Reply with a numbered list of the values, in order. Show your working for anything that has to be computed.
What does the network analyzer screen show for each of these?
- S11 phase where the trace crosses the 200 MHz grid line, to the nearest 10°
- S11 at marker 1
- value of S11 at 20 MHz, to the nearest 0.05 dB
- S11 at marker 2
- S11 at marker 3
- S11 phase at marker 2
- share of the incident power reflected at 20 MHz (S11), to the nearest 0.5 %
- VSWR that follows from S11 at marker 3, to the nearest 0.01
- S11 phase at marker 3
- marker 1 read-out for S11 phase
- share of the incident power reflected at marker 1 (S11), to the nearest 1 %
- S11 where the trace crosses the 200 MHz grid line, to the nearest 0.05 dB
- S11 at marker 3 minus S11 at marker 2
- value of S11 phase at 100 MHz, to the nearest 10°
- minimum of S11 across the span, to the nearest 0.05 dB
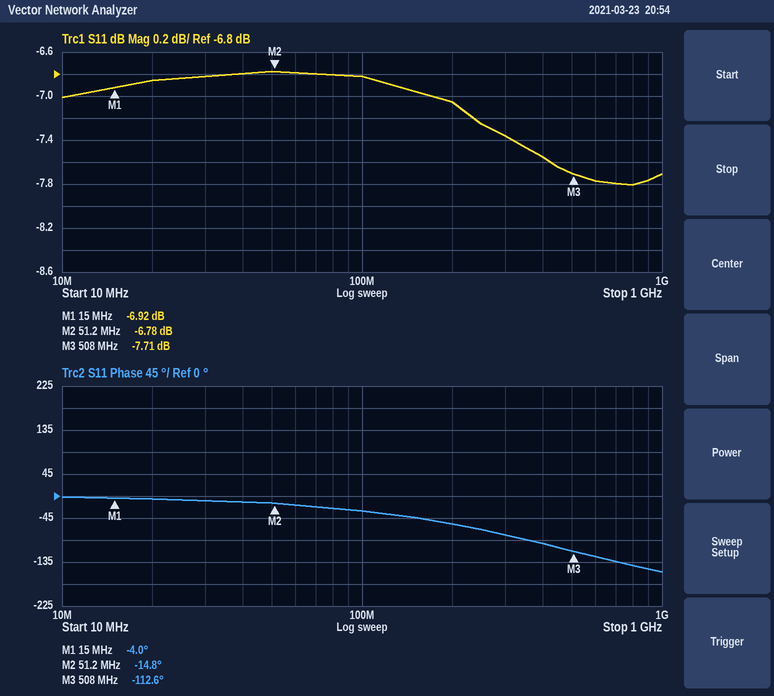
1. -60°
2. -6.92 dB
3. -6.85 dB
4. -6.78 dB
5. -7.71 dB
6. -14.8°
7. 10^(-6.85/10) ≈ 20.7 %, so 20.5 % to the nearest 0.5 %
8. (1 + 0.4116)/(1 − 0.4116) ≈ 2.40
9. -112.6°
10. -4.0°
11. 10^(-6.92/10) ≈ 20 %
12. -7.05 dB
13. -7.71 − (-6.78) = -0.93 dB
14. -30°
15. -7.80 dB
